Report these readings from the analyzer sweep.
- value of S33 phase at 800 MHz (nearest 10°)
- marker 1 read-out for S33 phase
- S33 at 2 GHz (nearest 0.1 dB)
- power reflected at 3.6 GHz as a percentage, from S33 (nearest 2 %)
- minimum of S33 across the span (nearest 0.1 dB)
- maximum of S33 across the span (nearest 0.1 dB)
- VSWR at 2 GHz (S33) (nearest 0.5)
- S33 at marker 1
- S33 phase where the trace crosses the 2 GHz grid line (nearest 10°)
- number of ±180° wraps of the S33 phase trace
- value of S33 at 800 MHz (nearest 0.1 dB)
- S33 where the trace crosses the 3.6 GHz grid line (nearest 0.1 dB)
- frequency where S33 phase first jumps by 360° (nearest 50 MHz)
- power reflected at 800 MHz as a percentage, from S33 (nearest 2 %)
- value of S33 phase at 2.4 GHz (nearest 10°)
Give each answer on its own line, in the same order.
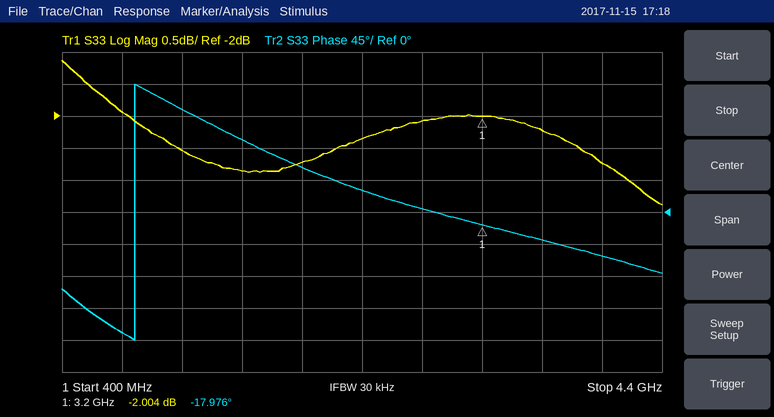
-170°
-17.976°
-2.7 dB
60 %
-3.4 dB
-1.1 dB
6.5
-2.004 dB
60°
1
-1.9 dB
-2.2 dB
900 MHz
64 %
30°
